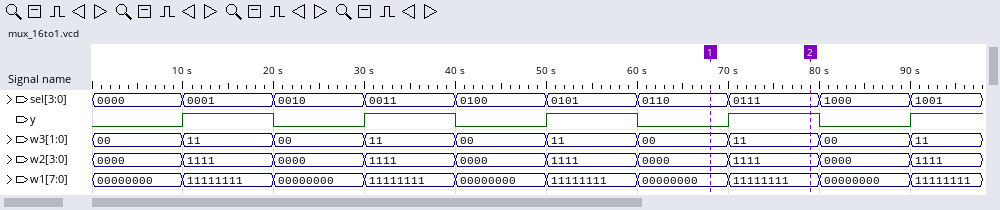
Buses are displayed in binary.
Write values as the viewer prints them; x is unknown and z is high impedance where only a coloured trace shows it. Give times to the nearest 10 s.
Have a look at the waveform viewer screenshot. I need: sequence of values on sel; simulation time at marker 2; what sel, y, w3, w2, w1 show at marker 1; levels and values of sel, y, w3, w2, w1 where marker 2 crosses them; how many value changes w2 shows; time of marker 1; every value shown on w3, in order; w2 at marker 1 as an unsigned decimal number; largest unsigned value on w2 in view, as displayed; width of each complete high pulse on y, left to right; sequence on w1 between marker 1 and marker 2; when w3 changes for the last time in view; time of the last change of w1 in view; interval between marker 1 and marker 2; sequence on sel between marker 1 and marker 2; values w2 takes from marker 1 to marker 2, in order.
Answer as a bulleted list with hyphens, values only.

- 0000, 0001, 0010, 0011, 0100, 0101, 0110, 0111, 1000, 1001
- 80 s
- sel=0110, y=0, w3=00, w2=0000, w1=00000000
- sel=0111, y=1, w3=11, w2=1111, w1=11111111
- 9
- 70 s
- 00, 11, 00, 11, 00, 11, 00, 11, 00, 11
- 0
- 1111
- 10 s, 10 s, 10 s, 10 s
- 00000000, 11111111
- 90 s
- 90 s
- 10 s
- 0110, 0111
- 0000, 1111
